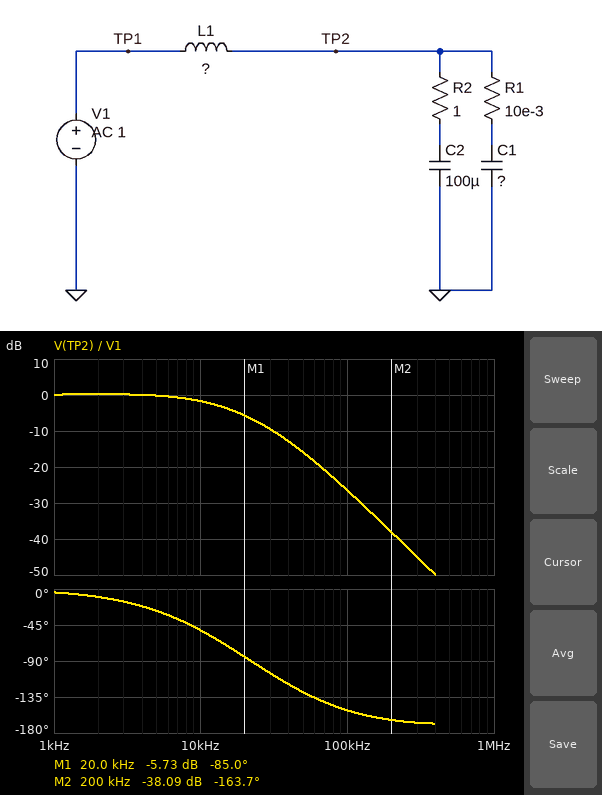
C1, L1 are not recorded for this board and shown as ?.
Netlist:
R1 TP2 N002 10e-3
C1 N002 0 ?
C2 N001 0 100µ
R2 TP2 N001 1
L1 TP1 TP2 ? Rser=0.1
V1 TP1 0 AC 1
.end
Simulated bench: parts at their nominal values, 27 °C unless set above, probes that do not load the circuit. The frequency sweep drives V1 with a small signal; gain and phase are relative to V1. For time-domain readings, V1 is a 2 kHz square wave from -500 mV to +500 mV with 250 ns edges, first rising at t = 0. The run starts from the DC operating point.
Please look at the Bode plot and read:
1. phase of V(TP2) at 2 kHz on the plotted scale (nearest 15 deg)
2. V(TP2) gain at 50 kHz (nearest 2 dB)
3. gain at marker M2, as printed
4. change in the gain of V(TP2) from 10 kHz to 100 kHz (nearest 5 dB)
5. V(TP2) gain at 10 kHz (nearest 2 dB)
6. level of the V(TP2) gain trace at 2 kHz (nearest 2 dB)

-15 deg
-16 dB
-38.09 dB
-25 dB
-2 dB
0 dB
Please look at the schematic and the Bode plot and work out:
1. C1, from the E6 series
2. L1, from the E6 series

3.3 µF
15 µH
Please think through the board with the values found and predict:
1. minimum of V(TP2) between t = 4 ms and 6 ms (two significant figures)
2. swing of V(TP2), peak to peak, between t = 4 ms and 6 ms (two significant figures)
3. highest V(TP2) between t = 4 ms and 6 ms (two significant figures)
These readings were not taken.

-530 mV
1.1 V
530 mV
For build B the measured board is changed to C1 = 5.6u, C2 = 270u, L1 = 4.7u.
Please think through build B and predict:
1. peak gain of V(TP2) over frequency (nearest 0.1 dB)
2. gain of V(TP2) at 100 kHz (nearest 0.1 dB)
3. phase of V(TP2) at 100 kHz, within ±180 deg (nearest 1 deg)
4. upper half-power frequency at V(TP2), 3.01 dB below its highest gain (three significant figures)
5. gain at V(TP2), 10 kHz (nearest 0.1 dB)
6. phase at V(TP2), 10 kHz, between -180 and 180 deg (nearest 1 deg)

0.6 dB
-20.0 dB
-158 deg
37.6 kHz
-0.3 dB
-19 deg
